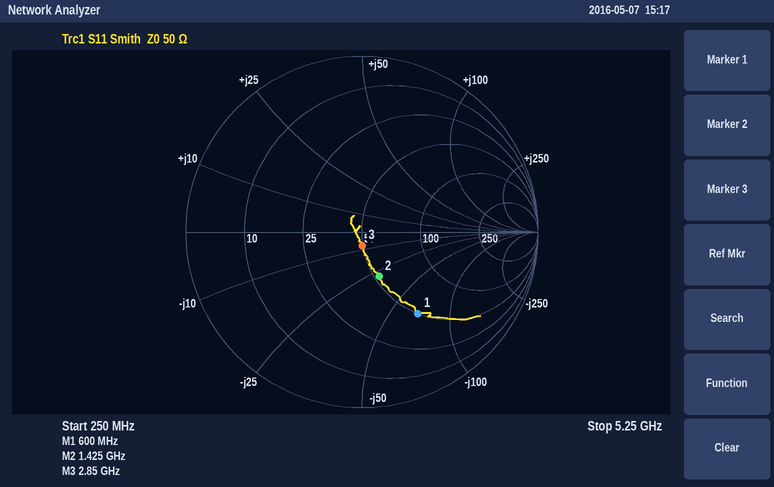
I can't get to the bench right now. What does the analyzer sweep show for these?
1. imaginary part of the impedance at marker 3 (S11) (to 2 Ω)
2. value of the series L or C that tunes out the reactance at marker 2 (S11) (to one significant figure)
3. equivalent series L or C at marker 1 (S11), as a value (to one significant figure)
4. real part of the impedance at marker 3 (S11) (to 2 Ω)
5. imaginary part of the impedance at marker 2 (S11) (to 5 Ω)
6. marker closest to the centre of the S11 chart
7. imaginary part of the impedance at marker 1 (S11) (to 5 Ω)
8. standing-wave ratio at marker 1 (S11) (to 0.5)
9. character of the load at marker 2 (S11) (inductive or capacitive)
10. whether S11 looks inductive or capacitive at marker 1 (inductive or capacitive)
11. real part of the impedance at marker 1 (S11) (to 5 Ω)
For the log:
-8 Ω
3 nH
4 pF
50 Ω
-30 Ω
marker 3
-70 Ω
3.5
capacitive
capacitive
50 Ω
